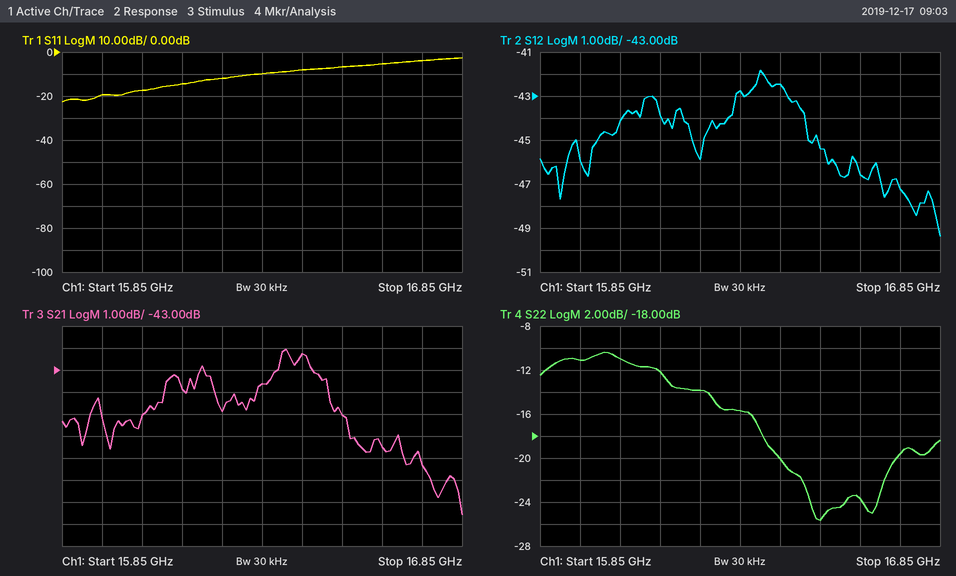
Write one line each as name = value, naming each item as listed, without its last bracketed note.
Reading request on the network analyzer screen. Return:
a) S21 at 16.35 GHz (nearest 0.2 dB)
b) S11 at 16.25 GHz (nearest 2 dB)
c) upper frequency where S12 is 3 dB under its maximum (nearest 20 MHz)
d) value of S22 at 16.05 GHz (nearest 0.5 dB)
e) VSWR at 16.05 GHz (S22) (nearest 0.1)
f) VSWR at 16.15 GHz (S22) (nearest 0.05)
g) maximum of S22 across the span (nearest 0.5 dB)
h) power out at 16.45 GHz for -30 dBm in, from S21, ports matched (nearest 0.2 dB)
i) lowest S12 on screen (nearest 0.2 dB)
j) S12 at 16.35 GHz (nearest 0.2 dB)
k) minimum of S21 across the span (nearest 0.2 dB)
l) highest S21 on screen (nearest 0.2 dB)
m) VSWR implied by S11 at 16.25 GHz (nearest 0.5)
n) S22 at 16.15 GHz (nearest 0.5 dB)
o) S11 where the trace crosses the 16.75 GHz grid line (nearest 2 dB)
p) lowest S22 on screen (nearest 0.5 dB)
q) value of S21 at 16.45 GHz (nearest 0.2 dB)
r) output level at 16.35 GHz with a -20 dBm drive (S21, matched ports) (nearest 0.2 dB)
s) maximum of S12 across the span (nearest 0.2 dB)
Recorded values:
S21 at 16.35 GHz = -43.6 dB
S11 at 16.25 GHz = -12 dB
upper frequency where S12 is 3 dB under its maximum = 16.52 GHz
value of S22 at 16.05 GHz = -11.0 dB
VSWR at 16.05 GHz (S22) = 1.8
VSWR at 16.15 GHz (S22) = 1.65
maximum of S22 across the span = -10.5 dB
power out at 16.45 GHz for -30 dBm in, from S21, ports matched = -72.2 dBm
lowest S12 on screen = -49.4 dB
S12 at 16.35 GHz = -42.8 dB
minimum of S21 across the span = -49.6 dB
highest S21 on screen = -42.0 dB
VSWR implied by S11 at 16.25 GHz = 1.5
S22 at 16.15 GHz = -12.0 dB
S11 where the trace crosses the 16.75 GHz grid line = -4 dB
lowest S22 on screen = -25.5 dB
value of S21 at 16.45 GHz = -42.2 dB
output level at 16.35 GHz with a -20 dBm drive (S21, matched ports) = -63.6 dBm
maximum of S12 across the span = -41.8 dB
